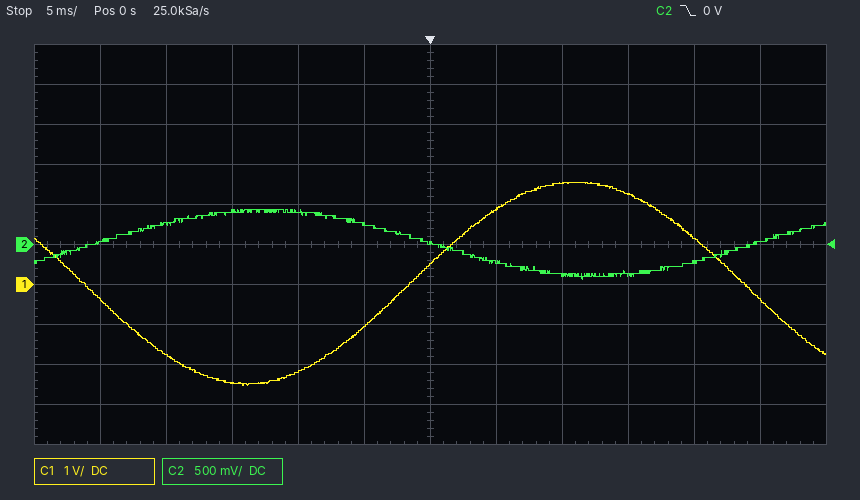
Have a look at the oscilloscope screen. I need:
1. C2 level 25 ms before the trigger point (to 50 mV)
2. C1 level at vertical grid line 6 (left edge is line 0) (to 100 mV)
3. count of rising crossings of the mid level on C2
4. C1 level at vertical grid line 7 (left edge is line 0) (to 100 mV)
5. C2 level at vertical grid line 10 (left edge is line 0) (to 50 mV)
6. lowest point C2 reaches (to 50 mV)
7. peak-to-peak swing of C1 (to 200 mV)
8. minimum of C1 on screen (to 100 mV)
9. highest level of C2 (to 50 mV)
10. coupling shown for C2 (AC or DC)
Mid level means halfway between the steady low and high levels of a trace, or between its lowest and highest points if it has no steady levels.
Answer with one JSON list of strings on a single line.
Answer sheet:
["50 mV", "500 mV", "2", "1.9 V", "-200 mV", "-450 mV", "5.0 V", "-2.5 V", "450 mV", "DC"]
